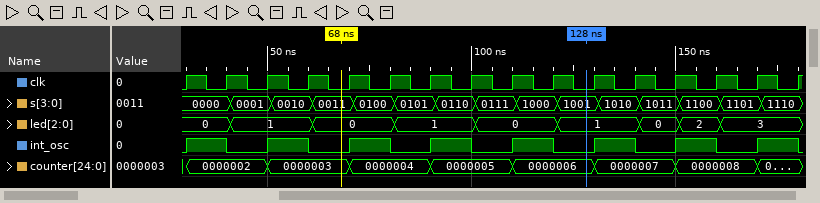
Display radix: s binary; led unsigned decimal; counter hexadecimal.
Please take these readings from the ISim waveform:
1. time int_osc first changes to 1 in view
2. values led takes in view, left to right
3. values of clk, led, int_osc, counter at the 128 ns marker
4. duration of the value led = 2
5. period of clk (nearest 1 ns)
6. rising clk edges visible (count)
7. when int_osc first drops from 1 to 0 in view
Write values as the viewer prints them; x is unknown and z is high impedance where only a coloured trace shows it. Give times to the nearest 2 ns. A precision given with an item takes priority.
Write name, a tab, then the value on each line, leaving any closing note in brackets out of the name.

time int_osc first changes to 1 in view	30 ns
values led takes in view, left to right	0, 1, 0, 1, 0, 1, 0, 2, 3
values of clk, led, int_osc, counter at the 128 ns marker	clk=0, led=1, int_osc=0, counter=0000006
duration of the value led = 2	10 ns
period of clk	10 ns
rising clk edges visible	16
when int_osc first drops from 1 to 0 in view	40 ns
